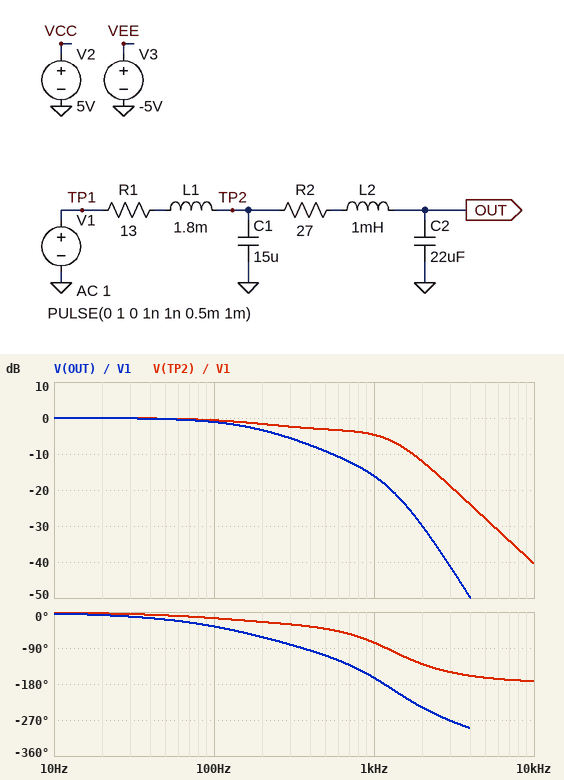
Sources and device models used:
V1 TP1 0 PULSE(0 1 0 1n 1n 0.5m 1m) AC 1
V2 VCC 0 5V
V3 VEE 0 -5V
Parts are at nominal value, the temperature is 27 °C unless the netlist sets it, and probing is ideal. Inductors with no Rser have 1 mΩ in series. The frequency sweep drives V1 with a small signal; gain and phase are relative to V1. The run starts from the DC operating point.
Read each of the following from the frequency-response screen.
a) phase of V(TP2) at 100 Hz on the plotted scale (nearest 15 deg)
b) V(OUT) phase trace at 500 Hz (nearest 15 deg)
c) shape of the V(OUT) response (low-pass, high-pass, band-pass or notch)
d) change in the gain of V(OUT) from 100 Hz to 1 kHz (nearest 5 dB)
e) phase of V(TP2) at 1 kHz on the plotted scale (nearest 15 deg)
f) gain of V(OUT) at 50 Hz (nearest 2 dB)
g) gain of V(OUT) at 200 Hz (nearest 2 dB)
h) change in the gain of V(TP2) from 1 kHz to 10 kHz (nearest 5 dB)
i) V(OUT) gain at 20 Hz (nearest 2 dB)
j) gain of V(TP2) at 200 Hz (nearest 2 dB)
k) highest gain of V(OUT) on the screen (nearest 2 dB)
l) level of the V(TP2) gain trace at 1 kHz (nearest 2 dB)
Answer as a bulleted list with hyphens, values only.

- -15 deg
- -105 deg
- low-pass
- -15 dB
- -75 deg
- 0 dB
- -4 dB
- -35 dB
- 0 dB
- -2 dB
- 0 dB
- -4 dB
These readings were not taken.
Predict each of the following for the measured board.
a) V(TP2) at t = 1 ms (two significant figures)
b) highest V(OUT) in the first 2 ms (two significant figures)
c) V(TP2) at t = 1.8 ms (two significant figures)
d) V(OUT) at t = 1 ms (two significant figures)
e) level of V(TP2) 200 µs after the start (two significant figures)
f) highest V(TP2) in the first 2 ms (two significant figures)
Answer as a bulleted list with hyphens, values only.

- 75 mV
- 540 mV
- 280 mV
- 330 mV
- 390 mV
- 850 mV
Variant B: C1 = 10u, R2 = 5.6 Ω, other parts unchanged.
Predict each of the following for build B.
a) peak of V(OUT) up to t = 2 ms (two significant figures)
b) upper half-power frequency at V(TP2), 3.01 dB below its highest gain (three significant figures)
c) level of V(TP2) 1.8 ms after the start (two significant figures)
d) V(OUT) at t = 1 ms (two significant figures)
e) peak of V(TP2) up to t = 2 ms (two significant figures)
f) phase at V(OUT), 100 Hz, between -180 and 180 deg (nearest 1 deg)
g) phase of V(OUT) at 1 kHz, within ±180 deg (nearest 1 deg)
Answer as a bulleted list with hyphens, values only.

- 710 mV
- 380 Hz
- 370 mV
- 350 mV
- 680 mV
- -19 deg
- -135 deg
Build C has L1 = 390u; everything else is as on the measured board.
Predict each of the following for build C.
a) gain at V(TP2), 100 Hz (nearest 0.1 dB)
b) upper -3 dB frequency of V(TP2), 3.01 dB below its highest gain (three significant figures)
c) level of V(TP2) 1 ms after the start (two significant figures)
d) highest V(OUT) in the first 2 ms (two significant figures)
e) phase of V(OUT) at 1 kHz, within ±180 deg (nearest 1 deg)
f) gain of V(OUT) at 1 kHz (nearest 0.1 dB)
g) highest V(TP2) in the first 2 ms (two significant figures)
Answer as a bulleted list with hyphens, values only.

- -0.8 dB
- 314 Hz
- 110 mV
- 520 mV
- -135 deg
- -16.7 dB
- 800 mV
